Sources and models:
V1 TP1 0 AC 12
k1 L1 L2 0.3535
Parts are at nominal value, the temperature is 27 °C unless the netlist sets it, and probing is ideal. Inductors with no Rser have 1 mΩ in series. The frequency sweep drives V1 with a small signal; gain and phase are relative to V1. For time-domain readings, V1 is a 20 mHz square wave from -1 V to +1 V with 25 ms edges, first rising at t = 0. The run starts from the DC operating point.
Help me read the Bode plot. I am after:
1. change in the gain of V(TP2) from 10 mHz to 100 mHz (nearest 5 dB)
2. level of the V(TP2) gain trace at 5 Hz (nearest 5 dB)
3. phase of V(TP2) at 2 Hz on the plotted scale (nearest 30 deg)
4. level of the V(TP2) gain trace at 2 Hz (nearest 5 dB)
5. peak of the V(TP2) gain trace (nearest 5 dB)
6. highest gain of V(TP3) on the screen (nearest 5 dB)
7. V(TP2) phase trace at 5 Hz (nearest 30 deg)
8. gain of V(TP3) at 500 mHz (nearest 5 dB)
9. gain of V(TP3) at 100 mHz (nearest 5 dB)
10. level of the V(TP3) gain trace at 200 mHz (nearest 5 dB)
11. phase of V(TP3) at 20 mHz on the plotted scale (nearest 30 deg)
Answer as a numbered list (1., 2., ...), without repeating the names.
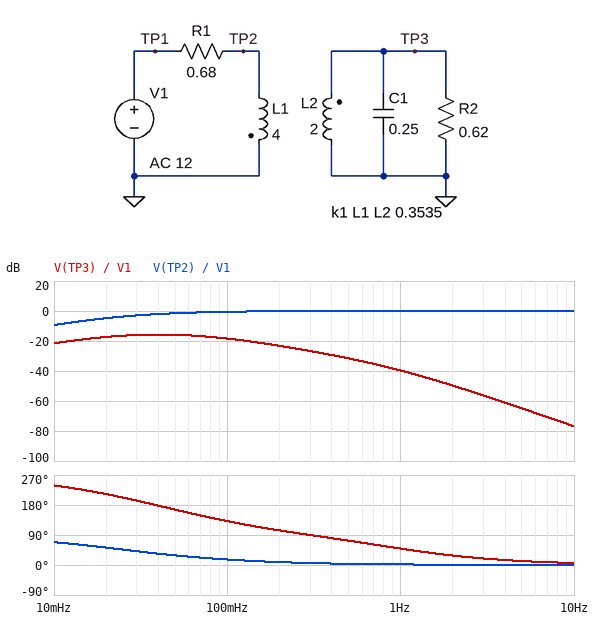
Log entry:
1. 10 dB
2. 0 dB
3. 0 deg
4. 0 dB
5. 0 dB
6. -15 dB
7. 0 deg
8. -30 dB
9. -20 dB
10. -25 dB
11. 210 deg
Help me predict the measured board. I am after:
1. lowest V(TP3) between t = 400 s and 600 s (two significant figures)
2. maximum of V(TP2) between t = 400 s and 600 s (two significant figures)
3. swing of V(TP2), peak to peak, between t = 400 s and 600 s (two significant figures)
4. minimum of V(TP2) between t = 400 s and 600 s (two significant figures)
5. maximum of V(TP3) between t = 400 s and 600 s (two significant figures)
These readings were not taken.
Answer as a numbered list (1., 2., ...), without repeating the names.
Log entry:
1. -240 mV
2. 2.0 V
3. 3.9 V
4. -2.0 V
5. 240 mV
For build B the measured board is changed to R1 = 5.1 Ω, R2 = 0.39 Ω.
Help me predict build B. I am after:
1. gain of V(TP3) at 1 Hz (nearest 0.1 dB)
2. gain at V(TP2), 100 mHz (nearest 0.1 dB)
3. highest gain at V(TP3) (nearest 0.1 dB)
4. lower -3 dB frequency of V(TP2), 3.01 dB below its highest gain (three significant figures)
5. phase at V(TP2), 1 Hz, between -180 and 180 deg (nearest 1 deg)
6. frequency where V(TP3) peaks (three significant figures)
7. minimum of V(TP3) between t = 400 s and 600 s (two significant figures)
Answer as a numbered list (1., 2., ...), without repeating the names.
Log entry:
1. -42.5 dB
2. -8.1 dB
3. -29.5 dB
4. 236 mHz
5. 13 deg
6. 85.3 mHz
7. -56 mV
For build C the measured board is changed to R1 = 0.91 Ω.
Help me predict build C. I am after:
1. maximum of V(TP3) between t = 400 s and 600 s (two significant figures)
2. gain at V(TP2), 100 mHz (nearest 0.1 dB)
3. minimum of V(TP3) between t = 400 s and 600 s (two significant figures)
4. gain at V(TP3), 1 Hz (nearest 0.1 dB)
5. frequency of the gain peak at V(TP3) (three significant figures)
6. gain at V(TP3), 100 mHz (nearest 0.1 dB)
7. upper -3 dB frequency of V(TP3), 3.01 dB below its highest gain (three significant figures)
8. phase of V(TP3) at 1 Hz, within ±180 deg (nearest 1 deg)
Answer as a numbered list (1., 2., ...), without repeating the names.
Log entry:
1. 220 mV
2. -0.8 dB
3. -220 mV
4. -39.7 dB
5. 46.5 mHz
6. -18.7 dB
7. 119 mHz
8. 50 deg
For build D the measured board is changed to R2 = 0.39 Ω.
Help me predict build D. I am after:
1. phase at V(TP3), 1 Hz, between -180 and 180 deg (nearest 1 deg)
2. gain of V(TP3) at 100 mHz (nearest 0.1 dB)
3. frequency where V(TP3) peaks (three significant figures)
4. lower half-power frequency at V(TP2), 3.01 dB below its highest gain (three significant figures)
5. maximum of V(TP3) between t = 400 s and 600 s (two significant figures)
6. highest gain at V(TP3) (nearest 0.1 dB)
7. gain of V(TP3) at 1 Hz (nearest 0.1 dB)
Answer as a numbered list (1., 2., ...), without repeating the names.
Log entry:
1. 62 deg
2. -21.9 dB
3. 31.4 mHz
4. 30.8 mHz
5. 190 mV
6. -17.4 dB
7. -42.3 dB
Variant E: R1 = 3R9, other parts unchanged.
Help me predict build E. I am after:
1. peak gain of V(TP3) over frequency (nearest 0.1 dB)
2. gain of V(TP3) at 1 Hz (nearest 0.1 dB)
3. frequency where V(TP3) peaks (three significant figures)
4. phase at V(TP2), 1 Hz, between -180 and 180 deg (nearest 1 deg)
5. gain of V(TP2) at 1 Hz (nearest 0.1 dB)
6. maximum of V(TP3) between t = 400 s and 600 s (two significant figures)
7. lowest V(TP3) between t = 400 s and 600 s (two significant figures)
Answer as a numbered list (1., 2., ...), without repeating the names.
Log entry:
1. -24.1 dB
2. -39.8 dB
3. 95.2 mHz
4. 10 deg
5. -0.1 dB
6. 98 mV
7. -98 mV
